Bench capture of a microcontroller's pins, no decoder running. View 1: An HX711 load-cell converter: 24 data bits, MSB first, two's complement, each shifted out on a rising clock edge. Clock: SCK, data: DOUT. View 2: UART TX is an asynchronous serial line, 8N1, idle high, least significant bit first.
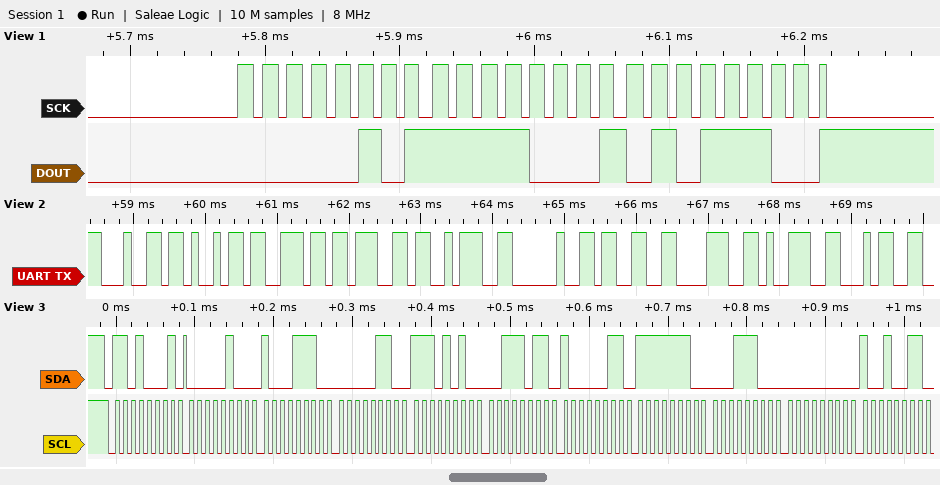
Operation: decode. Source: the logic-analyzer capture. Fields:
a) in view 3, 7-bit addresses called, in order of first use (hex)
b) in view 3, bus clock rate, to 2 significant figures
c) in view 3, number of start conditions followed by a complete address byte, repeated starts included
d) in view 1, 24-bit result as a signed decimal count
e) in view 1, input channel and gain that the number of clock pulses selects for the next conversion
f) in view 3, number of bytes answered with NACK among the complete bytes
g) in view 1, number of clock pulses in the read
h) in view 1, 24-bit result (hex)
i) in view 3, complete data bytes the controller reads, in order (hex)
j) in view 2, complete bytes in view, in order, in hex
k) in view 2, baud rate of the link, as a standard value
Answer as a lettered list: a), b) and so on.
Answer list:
a) 0x68
b) 100 kHz
c) 1
d) 389468
e) channel A, gain 128
f) 0
g) 25
h) 0x05F15C
i) 04 8E 06 EA 3B 83 FE 1C 00 93
j) 64 69 6E 67 3A 20 33 38 39 34
k) 9600 baud
